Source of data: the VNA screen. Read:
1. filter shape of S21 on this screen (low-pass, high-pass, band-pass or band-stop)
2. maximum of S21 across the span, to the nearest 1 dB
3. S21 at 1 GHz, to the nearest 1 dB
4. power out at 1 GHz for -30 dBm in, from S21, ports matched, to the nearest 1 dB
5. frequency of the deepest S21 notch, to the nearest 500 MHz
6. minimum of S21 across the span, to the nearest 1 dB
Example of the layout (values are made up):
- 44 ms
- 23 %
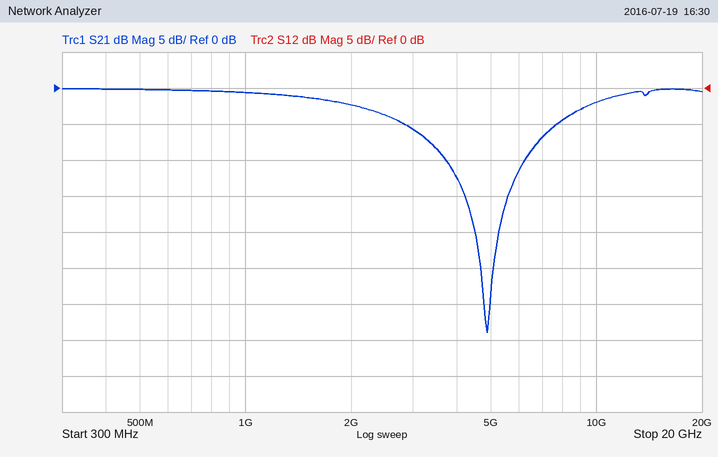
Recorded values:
- band-stop
- 0 dB
- -1 dB
- -31 dBm
- 5.0 GHz
- -34 dB
